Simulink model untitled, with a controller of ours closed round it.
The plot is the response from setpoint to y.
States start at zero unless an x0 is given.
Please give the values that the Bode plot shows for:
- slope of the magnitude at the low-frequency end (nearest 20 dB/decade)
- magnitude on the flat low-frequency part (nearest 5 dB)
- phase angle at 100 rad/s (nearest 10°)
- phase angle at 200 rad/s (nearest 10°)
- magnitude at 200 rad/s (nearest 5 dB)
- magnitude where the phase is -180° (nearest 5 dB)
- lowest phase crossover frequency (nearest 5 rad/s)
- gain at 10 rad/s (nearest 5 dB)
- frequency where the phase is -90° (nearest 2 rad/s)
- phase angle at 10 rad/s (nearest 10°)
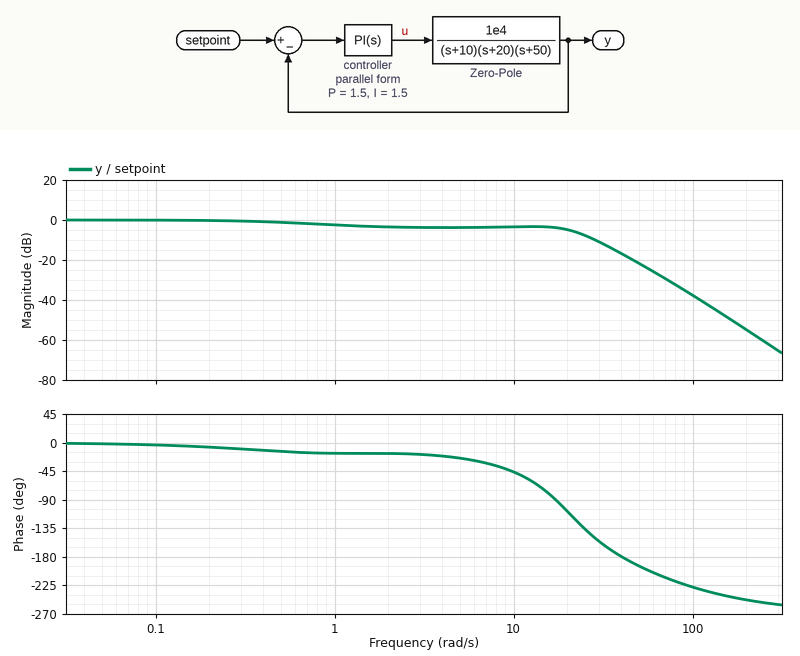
0 dB/decade
0 dB
-230°
-250°
-55 dB
-15 dB
40 rad/s
-5 dB
18 rad/s
-50°
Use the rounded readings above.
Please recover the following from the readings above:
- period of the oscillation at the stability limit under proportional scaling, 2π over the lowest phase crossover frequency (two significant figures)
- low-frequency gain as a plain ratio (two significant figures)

0.16 s
1.0
